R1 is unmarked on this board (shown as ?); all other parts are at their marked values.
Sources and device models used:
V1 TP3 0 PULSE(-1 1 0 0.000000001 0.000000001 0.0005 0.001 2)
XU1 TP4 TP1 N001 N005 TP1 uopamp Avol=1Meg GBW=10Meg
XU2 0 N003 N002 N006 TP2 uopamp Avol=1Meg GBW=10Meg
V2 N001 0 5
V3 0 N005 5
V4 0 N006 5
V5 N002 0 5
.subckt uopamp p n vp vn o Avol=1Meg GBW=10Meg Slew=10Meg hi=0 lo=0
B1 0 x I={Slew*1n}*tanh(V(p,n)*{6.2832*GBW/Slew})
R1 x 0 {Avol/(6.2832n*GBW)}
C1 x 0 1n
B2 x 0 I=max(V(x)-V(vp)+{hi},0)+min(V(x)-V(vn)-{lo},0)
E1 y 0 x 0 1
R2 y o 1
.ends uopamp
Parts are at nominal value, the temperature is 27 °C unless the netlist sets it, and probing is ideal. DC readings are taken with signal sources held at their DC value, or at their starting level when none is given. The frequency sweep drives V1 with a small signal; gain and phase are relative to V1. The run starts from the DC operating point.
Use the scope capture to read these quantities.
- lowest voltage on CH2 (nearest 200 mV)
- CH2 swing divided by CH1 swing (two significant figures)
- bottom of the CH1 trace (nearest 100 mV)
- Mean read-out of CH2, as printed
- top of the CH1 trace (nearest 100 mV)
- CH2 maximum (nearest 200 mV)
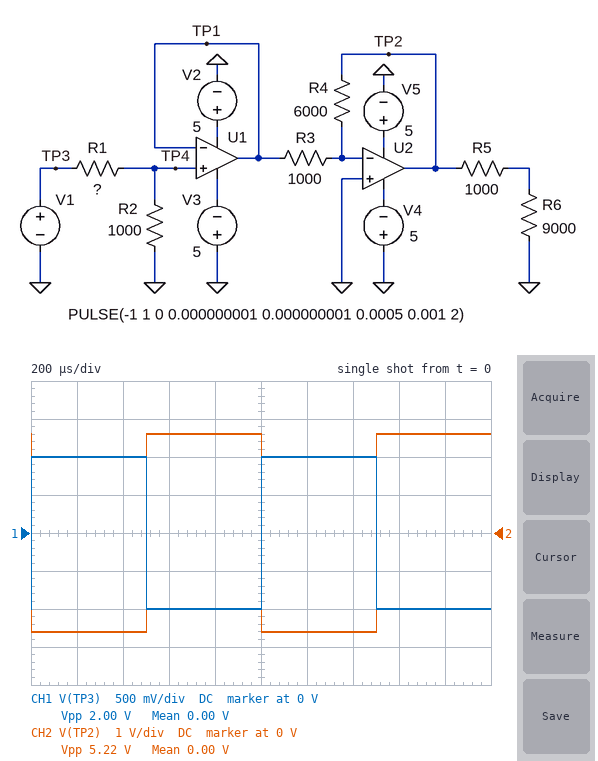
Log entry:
-2.6 V
2.6
-1.0 V
0.00 V
1.0 V
2.6 V
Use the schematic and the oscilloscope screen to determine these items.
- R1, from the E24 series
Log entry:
1.3 kΩ
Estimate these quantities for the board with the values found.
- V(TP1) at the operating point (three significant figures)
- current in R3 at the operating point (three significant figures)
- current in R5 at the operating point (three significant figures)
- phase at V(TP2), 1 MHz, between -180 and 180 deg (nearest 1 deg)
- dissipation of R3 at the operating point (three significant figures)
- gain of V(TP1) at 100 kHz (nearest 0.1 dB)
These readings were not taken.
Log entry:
-435 mV
435 µA
261 µA
139 deg
189 µW
-7.2 dB
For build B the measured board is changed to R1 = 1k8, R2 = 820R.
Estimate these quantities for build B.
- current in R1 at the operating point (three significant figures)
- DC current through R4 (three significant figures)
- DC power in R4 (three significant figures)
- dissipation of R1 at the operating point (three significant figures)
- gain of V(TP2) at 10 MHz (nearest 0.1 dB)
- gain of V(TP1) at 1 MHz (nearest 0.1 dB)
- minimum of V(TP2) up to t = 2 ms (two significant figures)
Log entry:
382 µA
313 µA
588 µW
262 µW
-14.5 dB
-10.1 dB
-1.9 V
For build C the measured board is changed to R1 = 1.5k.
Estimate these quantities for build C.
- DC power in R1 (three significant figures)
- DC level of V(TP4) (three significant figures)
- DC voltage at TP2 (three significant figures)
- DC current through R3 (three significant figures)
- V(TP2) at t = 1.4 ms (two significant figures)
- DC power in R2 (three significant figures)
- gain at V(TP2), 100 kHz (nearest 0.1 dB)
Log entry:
240 µW
-400 mV
2.40 V
400 µA
-2.4 V
160 µW
7.6 dB
